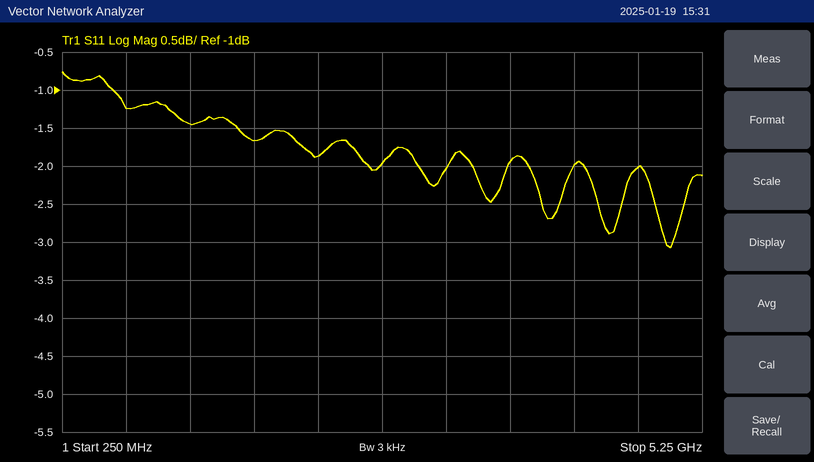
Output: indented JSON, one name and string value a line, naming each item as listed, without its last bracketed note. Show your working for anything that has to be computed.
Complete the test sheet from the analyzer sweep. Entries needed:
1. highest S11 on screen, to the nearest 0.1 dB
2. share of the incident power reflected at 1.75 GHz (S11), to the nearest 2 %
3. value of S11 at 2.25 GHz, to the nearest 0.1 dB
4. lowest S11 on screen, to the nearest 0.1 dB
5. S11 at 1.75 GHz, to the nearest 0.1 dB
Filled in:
{
  "highest S11 on screen, to the nearest 0.1 dB": "-0.8 dB",
  "share of the incident power reflected at 1.75 GHz (S11), to the nearest 2 %": "10^(-1.7/10) ≈ 68 %",
  "value of S11 at 2.25 GHz, to the nearest 0.1 dB": "-1.9 dB",
  "lowest S11 on screen, to the nearest 0.1 dB": "-3.1 dB",
  "S11 at 1.75 GHz, to the nearest 0.1 dB": "-1.7 dB"
}
